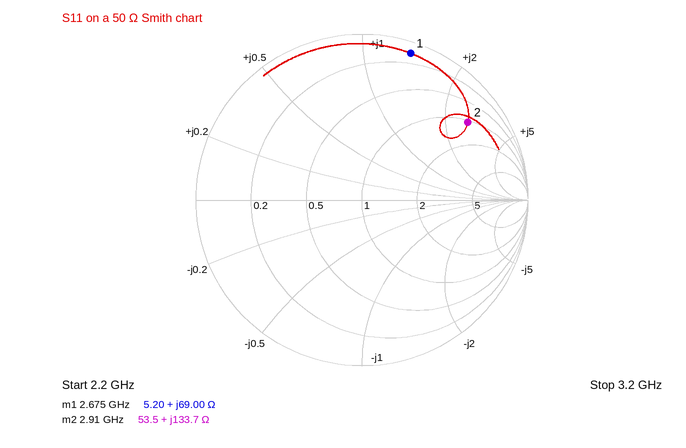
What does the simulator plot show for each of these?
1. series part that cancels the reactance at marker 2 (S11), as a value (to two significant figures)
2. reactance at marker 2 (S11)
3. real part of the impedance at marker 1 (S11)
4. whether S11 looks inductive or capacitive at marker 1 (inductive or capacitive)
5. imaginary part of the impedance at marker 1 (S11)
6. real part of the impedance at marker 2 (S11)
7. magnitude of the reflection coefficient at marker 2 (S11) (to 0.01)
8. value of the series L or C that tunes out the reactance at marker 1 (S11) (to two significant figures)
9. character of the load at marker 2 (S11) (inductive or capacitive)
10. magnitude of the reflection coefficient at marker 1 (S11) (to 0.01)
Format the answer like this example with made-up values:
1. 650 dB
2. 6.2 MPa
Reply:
1. 410 fF
2. +133.7 Ω
3. 5.20 Ω
4. inductive
5. +69.00 Ω
6. 53.5 Ω
7. 0.79
8. 860 fF
9. inductive
10. 0.93
